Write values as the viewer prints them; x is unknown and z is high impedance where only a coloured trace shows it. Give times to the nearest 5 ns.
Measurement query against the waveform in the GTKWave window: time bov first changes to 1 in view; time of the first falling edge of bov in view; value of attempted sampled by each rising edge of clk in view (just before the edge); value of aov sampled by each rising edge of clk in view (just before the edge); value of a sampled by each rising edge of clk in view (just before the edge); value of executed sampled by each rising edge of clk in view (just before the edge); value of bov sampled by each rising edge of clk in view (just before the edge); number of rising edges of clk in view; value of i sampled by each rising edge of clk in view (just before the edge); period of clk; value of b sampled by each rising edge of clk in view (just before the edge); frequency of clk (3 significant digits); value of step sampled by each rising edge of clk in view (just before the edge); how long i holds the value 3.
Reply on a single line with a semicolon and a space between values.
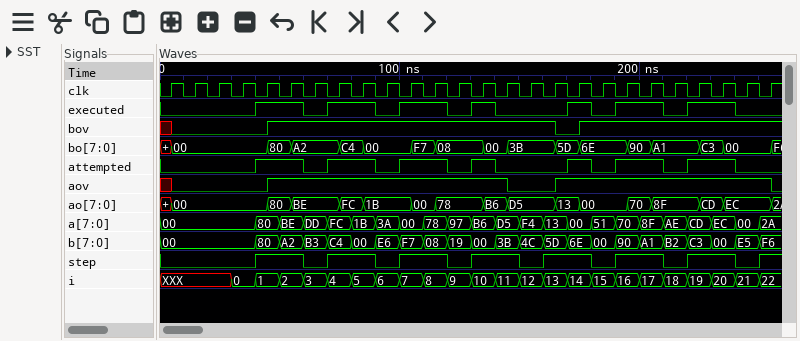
45 ns; 165 ns; 0 0 0 0 1 1 0 1 1 0 1 1 0 1 0 0 0 1 0 1 1 0 1 1 0 0; x 0 0 0 0 1 1 1 1 1 1 1 1 1 1 0 0 1 1 1 1 1 1 1 1 1; 00, 00, 00, 00, 80, BE, DD, FC, 1B, 3A, 00, 78, 97, B6, D5, F4, 13, 00, 51, 70, 8F, AE, CD, EC, 00, 2A; 0 0 0 0 1 1 0 1 1 0 1 1 0 1 0 0 0 1 0 1 1 0 1 1 0 0; x 0 0 0 0 1 1 1 1 1 1 1 1 1 1 1 1 0 1 1 1 1 1 1 1 1; 26; XXX, XXX, XXX, 0, 1, 2, 3, 4, 5, 6, 7, 8, 9, 10, 11, 12, 13, 14, 15, 16, 17, 18, 19, 20, 21, 22; 10 ns; 00, 00, 00, 00, 80, A2, B3, C4, 00, E6, F7, 08, 19, 00, 3B, 4C, 5D, 6E, 00, 90, A1, B2, C3, 00, E5, F6; 100 MHz; 0 0 0 0 1 1 0 1 1 0 1 1 0 1 1 0 1 1 0 1 1 0 1 1 0 1; 10 ns
